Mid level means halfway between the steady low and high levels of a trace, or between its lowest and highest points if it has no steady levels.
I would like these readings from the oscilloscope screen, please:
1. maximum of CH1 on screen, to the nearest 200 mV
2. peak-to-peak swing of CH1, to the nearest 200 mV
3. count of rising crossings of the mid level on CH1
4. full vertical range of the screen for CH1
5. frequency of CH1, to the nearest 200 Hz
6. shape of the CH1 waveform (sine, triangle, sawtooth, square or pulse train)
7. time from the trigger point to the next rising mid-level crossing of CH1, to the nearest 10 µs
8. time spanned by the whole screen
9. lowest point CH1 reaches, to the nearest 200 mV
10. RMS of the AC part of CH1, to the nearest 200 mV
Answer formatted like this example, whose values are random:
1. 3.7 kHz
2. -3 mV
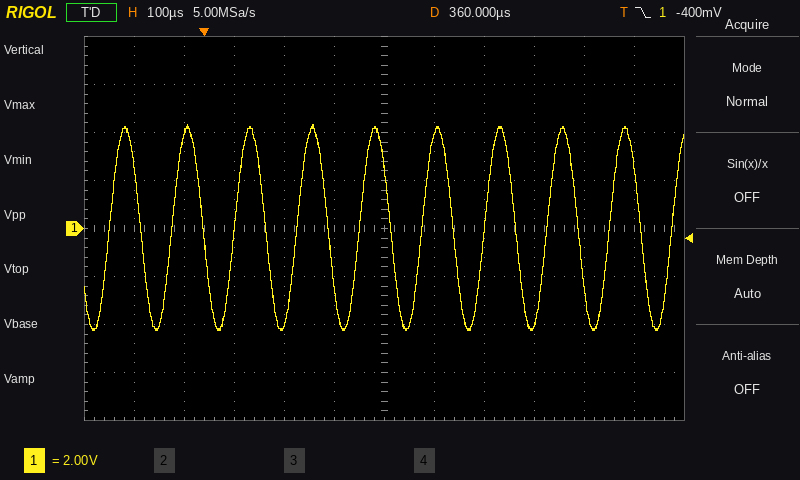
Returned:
1. 4.4 V
2. 8.6 V
3. 10
4. 16 V
5. 8.0 kHz
6. sine
7. 60 µs
8. 1.2 ms
9. -4.2 V
10. 3.0 V
